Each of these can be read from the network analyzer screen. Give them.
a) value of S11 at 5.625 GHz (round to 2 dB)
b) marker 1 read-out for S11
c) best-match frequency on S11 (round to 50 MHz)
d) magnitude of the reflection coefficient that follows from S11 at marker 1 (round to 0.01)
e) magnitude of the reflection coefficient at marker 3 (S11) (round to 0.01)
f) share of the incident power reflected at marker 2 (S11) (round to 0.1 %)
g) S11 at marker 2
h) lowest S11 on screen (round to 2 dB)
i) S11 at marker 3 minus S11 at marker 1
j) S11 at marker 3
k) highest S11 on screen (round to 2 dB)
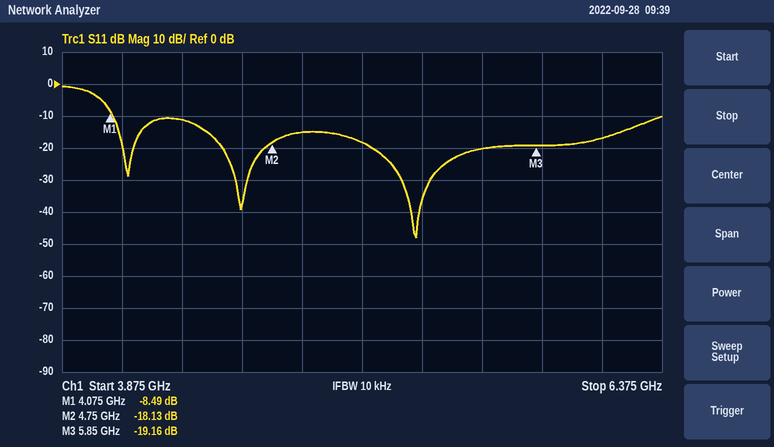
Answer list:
-20 dB
-8.49 dB
5.35 GHz
0.38
0.11
1.5 %
-18.13 dB
-48 dB
-10.67 dB
-19.16 dB
0 dB
